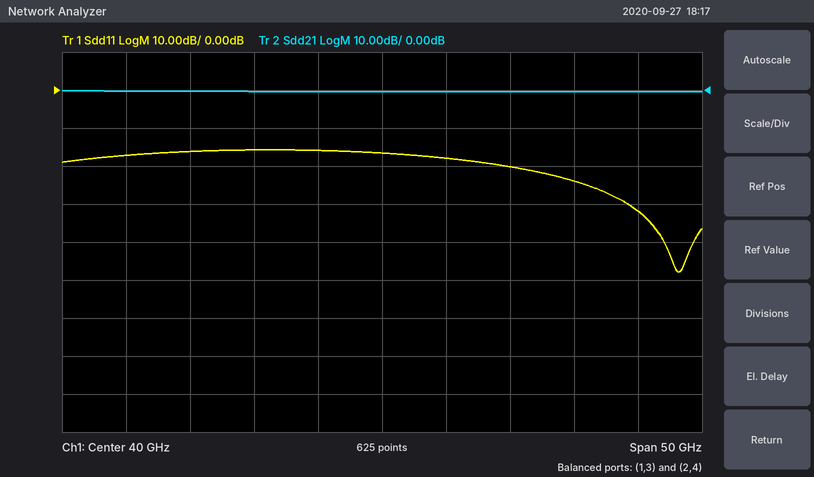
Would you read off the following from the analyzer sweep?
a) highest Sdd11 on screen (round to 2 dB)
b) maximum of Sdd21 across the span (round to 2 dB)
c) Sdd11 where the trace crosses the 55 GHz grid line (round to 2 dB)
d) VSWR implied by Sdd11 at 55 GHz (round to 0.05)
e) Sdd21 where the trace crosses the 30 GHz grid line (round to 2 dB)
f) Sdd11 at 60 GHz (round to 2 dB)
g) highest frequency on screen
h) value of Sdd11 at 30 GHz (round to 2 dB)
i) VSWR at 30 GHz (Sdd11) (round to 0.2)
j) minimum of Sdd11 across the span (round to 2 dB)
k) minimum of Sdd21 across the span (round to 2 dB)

-16 dB
0 dB
-24 dB
1.15
0 dB
-32 dB
65 GHz
-16 dB
1.4
-48 dB
0 dB
